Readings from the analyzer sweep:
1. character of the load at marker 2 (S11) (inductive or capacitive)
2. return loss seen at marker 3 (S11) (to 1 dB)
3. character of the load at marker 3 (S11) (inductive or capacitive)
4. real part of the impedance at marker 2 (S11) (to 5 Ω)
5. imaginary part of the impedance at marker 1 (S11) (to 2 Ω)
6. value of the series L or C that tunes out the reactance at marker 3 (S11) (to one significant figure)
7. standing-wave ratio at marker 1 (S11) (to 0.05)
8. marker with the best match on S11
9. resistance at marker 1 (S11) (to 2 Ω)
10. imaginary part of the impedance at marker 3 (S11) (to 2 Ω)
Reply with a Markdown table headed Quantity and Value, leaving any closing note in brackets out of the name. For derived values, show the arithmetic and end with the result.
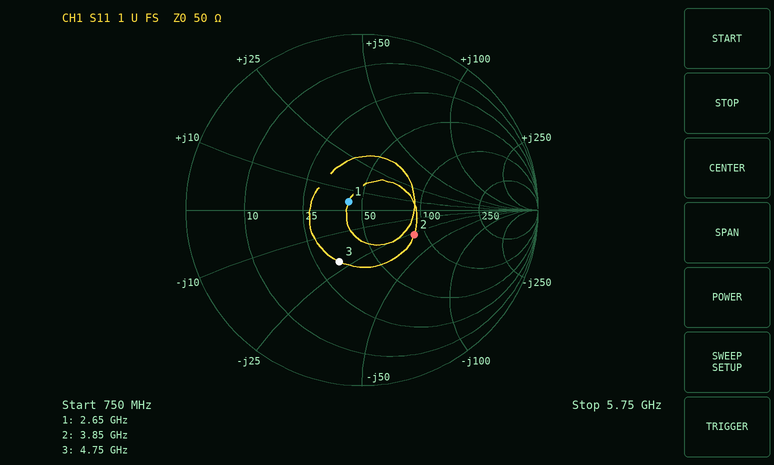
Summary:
| Quantity | Value |
|---|---|
| character of the load at marker 2 (S11) | capacitive |
| return loss seen at marker 3 (S11) | 10 dB |
| character of the load at marker 3 (S11) | capacitive |
| real part of the impedance at marker 2 (S11) | 85 Ω |
| imaginary part of the impedance at marker 1 (S11) | +4 Ω |
| value of the series L or C that tunes out the reactance at marker 3 (S11) | L = 22 Ω/(2π × 4.75 GHz) ≈ 737 pH, so 700 pH to one significant figure |
| standing-wave ratio at marker 1 (S11) | 1.20 |
| marker with the best match on S11 | marker 1 |
| resistance at marker 1 (S11) | 42 Ω |
| imaginary part of the impedance at marker 3 (S11) | -22 Ω |
